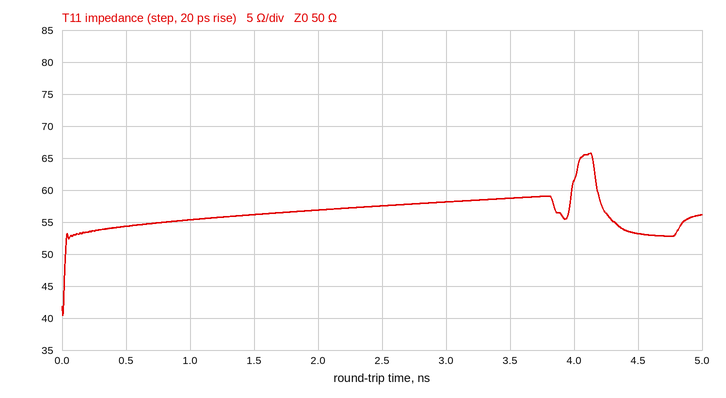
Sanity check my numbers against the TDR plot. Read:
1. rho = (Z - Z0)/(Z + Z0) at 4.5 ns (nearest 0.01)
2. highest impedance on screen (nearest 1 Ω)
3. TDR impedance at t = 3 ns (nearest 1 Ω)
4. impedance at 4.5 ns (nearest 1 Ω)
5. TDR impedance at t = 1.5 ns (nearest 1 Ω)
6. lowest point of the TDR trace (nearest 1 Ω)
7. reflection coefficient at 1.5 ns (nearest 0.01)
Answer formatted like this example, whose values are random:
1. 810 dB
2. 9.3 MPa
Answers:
1. +0.03
2. 66 Ω
3. 58 Ω
4. 53 Ω
5. 56 Ω
6. 40 Ω
7. +0.06
